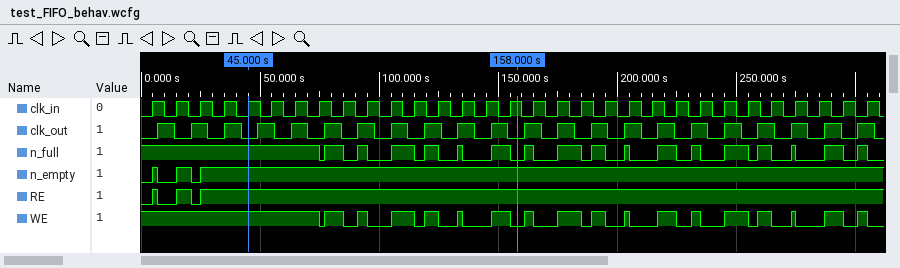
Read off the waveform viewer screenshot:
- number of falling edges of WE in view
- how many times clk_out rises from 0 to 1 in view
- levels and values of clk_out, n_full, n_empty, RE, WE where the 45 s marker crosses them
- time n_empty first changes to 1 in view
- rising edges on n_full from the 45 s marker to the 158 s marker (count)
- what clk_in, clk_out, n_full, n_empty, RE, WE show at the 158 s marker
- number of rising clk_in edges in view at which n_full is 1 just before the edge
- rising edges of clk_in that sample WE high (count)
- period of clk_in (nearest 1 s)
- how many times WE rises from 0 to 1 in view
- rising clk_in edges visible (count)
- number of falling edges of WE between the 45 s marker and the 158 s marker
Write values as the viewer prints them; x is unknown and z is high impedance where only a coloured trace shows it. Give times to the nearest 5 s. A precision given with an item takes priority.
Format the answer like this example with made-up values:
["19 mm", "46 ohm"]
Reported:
["18", "22", "clk_out=0, n_full=1, n_empty=1, RE=1, WE=1", "5 s", "6", "clk_in=1, clk_out=0, n_full=0, n_empty=1, RE=1, WE=0", "25", "25", "10 s", "17", "31", "7"]
